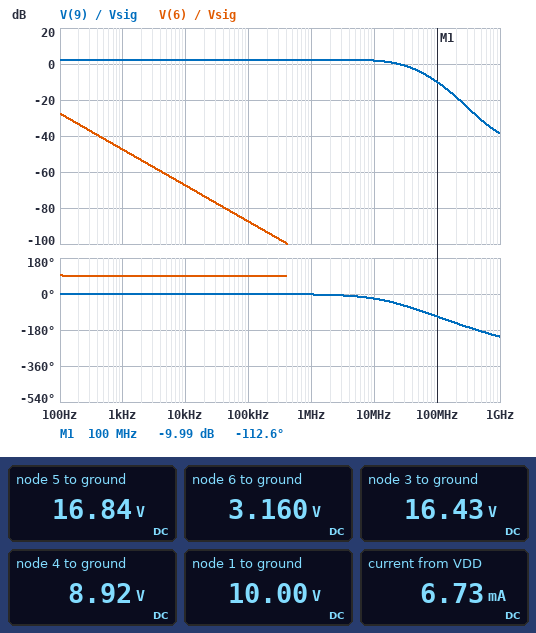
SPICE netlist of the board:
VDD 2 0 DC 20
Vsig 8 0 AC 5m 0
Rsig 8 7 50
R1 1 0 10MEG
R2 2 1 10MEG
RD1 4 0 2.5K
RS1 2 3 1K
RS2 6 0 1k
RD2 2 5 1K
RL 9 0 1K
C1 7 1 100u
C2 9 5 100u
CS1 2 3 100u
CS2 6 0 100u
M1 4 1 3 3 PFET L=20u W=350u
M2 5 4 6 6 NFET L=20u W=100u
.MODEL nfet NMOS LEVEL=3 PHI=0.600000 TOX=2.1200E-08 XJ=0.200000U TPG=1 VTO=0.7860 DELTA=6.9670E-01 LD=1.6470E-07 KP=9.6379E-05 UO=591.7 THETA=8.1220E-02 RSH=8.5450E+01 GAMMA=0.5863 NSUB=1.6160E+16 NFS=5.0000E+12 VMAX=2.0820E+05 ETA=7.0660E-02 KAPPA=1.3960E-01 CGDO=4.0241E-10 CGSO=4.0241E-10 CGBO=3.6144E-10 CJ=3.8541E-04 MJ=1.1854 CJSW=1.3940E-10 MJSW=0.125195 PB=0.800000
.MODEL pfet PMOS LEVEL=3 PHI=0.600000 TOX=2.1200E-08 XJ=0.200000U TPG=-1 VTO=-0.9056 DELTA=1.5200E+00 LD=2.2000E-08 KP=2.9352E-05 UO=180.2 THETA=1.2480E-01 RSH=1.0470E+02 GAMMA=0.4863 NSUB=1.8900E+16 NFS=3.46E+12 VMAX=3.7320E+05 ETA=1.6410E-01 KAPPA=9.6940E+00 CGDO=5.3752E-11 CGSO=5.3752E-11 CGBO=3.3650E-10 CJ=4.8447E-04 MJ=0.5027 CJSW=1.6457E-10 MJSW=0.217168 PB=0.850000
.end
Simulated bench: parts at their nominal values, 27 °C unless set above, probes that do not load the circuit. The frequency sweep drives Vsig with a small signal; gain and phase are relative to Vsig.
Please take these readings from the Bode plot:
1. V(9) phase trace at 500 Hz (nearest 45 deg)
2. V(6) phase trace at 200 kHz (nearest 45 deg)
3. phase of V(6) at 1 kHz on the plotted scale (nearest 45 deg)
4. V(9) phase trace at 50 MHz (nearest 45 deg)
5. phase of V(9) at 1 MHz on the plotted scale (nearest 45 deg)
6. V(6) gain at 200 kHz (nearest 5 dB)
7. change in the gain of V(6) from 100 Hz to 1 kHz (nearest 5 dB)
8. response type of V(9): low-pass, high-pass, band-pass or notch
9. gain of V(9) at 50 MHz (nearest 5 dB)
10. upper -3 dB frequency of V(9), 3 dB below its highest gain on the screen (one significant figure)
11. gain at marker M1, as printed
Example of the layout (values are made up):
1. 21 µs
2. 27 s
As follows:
1. 0 deg
2. 90 deg
3. 90 deg
4. -90 deg
5. 0 deg
6. -95 dB
7. -20 dB
8. low-pass
9. -5 dB
10. 30 MHz
11. -9.99 dB
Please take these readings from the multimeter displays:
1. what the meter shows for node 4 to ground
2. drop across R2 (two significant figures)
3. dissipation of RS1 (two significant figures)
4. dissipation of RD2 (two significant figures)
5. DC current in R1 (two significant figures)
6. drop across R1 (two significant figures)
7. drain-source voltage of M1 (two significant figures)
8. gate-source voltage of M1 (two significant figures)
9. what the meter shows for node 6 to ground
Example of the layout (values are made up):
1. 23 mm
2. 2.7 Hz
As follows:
1. 8.92 V
2. 10 V
3. 13 mW
4. 10 mW
5. 1.0 µA
6. 10 V
7. -7.5 V
8. -6.4 V
9. 3.160 V
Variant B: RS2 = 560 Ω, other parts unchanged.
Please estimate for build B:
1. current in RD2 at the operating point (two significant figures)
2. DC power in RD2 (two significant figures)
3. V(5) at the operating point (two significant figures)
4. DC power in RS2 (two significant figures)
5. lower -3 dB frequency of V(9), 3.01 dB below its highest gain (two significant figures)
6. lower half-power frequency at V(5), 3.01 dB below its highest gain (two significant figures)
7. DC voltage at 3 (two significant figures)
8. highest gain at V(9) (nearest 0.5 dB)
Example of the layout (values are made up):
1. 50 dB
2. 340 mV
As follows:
1. 4.1 mA
2. 17 mW
3. 16 V
4. 9.4 mW
5. 4.6 Hz
6. 4.0 Hz
7. 16 V
8. 3.0 dB
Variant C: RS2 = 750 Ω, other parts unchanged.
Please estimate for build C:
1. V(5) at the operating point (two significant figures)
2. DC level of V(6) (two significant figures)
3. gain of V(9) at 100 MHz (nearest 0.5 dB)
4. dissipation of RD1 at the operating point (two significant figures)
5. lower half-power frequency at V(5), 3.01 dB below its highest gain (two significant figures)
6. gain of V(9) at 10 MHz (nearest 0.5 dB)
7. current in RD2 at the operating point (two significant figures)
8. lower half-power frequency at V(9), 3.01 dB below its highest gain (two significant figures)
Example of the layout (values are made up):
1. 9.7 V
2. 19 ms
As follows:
1. 16 V
2. 2.7 V
3. -9.5 dB
4. 32 mW
5. 3.8 Hz
6. 2.5 dB
7. 3.6 mA
8. 4.4 Hz
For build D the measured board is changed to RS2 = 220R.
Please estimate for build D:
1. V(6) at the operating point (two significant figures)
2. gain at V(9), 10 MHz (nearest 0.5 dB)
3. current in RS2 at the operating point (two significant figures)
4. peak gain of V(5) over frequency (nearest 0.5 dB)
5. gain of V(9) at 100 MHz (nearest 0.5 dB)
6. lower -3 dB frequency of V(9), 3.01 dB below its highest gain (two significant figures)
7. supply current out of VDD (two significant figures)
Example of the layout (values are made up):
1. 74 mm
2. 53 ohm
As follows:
1. 1.2 V
2. 3.5 dB
3. 5.4 mA
4. 4.0 dB
5. -8.5 dB
6. 4.5 Hz
7. 9.0 mA
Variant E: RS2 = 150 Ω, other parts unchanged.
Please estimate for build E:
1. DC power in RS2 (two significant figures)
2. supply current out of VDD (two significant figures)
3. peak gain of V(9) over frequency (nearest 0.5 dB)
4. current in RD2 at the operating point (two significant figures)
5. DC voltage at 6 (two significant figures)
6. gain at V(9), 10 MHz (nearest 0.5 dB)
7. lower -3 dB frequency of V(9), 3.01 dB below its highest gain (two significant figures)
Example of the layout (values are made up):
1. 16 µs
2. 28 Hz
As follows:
1. 5.1 mW
2. 9.4 mA
3. 4.0 dB
4. 5.8 mA
5. 870 mV
6. 3.5 dB
7. 4.0 Hz
